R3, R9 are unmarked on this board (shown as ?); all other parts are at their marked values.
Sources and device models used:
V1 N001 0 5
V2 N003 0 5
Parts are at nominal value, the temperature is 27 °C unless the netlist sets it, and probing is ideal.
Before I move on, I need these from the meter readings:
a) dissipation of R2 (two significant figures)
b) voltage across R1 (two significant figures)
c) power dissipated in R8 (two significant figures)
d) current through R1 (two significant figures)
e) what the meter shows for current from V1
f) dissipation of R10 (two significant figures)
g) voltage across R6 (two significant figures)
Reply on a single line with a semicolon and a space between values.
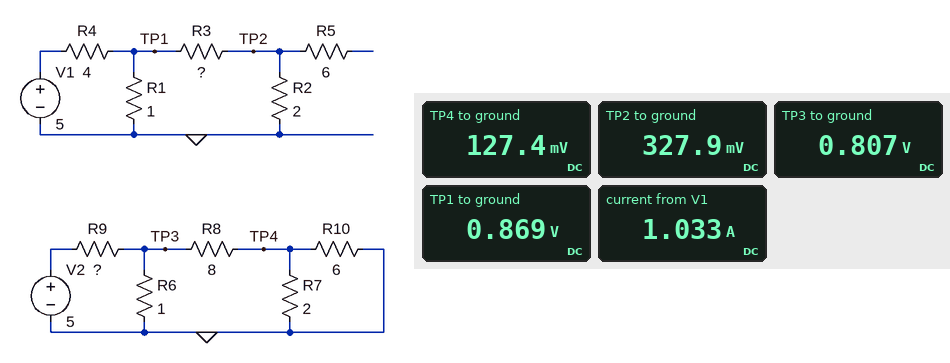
54 mW; 870 mV; 58 mW; 870 mA; 1.033 A; 2.7 mW; 810 mV
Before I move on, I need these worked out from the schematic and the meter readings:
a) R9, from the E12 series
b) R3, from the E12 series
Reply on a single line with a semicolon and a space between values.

4.7 Ω; 3.3 Ω
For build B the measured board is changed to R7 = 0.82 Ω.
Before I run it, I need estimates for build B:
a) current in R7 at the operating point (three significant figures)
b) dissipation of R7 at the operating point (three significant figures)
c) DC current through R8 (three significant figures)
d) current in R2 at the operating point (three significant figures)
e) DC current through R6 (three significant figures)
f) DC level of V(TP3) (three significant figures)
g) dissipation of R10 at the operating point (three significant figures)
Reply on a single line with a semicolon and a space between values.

80.8 mA; 5.36 mW; 91.9 mA; 164 mA; 801 mA; 801 mV; 732 µW
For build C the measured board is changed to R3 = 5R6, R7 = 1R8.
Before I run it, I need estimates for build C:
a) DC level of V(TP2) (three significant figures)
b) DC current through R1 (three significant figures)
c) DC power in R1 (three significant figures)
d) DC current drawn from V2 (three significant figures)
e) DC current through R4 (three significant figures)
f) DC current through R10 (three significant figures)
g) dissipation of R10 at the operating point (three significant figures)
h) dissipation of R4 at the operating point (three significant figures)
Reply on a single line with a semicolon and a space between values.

238 mV; 905 mA; 819 mW; 892 mA; 1.02 A; 19.8 mA; 2.36 mW; 4.19 W
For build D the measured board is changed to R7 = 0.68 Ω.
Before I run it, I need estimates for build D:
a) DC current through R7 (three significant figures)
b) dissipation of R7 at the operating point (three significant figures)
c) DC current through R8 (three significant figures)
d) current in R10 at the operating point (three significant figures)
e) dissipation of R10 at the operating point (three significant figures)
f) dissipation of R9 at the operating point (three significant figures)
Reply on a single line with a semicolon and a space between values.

83.5 mA; 4.74 mW; 93.0 mA; 9.46 mA; 537 µW; 3.75 W
